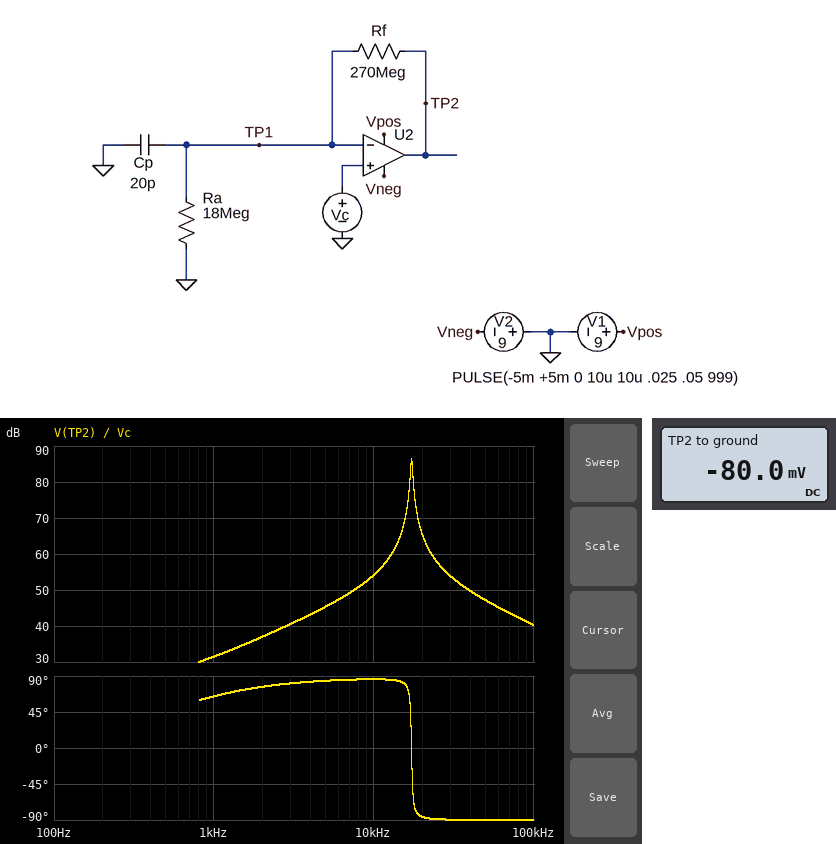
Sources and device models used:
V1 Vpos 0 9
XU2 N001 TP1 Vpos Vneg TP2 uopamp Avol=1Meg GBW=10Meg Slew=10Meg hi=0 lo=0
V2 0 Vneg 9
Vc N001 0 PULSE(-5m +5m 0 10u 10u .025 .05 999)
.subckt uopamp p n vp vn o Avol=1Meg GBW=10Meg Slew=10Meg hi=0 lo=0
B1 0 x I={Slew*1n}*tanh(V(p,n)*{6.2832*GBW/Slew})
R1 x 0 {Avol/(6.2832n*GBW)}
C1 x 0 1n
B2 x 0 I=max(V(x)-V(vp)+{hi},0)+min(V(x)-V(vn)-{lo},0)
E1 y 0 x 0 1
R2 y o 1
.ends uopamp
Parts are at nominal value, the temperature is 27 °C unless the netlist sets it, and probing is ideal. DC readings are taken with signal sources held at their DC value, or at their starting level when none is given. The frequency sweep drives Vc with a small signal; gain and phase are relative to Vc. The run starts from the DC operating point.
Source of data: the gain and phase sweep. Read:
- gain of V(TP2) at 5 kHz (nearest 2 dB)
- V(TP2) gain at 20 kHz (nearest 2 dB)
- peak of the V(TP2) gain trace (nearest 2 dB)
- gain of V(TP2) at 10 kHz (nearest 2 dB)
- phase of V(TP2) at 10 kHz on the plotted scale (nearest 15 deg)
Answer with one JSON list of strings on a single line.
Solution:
["46 dB", "66 dB", "86 dB", "54 dB", "90 deg"]
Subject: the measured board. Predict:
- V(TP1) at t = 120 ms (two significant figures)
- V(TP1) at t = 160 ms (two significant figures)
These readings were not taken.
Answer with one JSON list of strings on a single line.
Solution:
["5.0 mV", "5.0 mV"]
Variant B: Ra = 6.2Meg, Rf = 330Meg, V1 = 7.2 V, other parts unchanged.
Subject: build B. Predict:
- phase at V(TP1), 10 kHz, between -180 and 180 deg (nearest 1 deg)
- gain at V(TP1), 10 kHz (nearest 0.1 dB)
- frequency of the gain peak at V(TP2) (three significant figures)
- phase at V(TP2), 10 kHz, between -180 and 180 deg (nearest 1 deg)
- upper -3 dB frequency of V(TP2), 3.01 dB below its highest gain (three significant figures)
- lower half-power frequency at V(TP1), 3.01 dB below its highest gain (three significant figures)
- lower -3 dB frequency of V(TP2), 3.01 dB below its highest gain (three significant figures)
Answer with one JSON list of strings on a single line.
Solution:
["-5 deg", "4.6 dB", "15.5 kHz", "77 deg", "16.2 kHz", "14.8 kHz", "14.9 kHz"]
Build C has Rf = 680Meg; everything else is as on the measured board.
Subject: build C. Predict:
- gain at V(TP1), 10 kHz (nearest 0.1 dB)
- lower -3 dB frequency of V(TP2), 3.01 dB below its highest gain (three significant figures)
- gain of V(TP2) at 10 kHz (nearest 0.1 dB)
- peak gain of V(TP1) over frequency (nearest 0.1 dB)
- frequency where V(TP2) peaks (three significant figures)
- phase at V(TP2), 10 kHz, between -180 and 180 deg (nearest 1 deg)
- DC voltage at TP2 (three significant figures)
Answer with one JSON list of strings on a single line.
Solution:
["16.4 dB", "10.6 kHz", "75.1 dB", "27.4 dB", "10.8 kHz", "72 deg", "-194 mV"]
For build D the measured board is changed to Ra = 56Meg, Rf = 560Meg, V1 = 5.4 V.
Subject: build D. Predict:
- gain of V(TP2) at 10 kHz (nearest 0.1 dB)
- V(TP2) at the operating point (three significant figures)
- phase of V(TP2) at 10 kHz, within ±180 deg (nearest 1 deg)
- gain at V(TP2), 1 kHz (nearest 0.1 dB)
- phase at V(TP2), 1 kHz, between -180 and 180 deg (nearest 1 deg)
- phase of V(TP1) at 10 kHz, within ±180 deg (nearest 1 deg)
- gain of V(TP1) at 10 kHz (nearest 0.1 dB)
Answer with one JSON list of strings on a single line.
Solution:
["67.5 dB", "-55.0 mV", "87 deg", "37.1 dB", "81 deg", "-2 deg", "10.6 dB"]
